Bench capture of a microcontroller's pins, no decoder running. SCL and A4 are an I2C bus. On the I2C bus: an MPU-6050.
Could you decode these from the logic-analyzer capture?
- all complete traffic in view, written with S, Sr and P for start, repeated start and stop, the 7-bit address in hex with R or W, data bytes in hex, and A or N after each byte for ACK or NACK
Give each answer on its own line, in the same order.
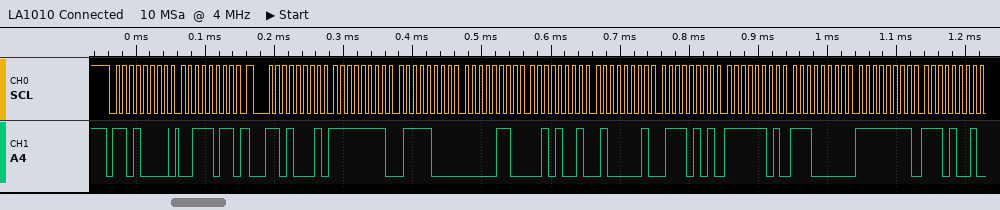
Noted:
S 68W A 3B A Sr 68R A FF A 78 A 06 A 29 A 41 A 75 A FD A E0 A FF A E9 A
